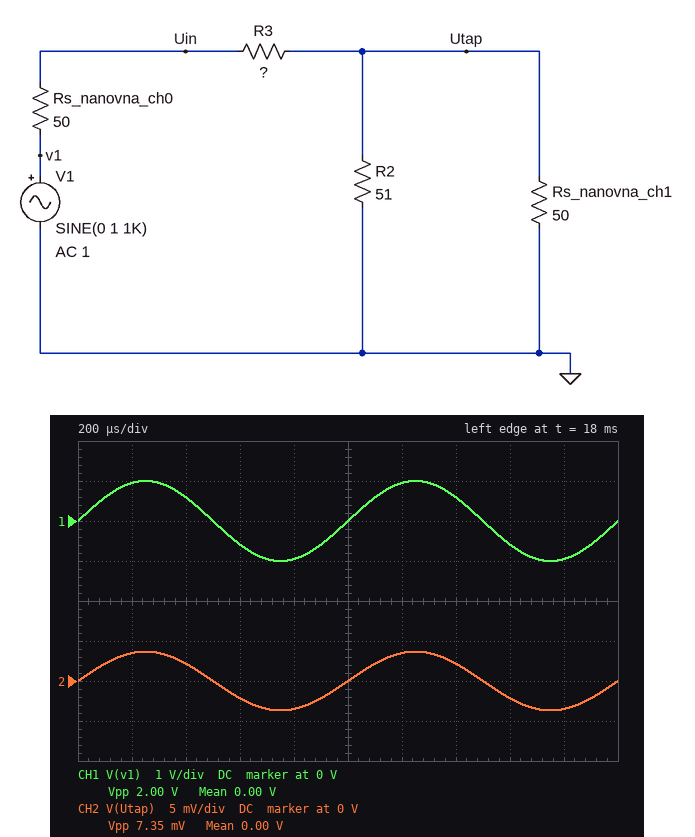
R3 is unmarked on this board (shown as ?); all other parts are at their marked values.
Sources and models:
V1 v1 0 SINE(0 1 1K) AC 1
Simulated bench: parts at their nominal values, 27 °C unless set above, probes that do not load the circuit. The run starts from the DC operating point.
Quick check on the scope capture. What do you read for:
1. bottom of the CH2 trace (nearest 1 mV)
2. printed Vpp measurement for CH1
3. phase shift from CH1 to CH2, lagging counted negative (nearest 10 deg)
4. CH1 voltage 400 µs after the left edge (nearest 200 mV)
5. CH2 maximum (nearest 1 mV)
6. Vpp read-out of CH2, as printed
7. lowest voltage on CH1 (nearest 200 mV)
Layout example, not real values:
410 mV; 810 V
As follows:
-4 mV; 2.00 V; 0 deg; 600 mV; 4 mV; 7.35 mV; -1.0 V
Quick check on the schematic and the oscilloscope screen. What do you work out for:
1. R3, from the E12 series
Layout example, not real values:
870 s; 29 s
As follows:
6.8 kΩ
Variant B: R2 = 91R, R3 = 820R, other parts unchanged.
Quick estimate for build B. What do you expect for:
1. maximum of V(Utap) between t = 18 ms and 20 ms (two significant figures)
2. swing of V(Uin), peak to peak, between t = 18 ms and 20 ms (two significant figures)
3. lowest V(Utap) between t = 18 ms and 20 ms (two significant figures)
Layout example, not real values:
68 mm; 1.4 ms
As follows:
36 mV; 1.9 V; -36 mV
